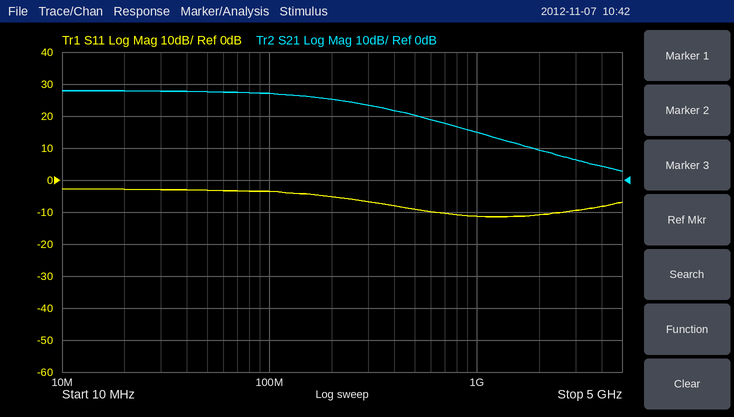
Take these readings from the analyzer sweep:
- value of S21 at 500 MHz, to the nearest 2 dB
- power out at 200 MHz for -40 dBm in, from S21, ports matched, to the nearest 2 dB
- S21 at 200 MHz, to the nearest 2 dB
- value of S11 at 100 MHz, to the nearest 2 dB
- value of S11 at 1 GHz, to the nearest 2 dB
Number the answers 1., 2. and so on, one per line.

1. 20 dB
2. -14 dBm
3. 26 dB
4. -4 dB
5. -12 dB
